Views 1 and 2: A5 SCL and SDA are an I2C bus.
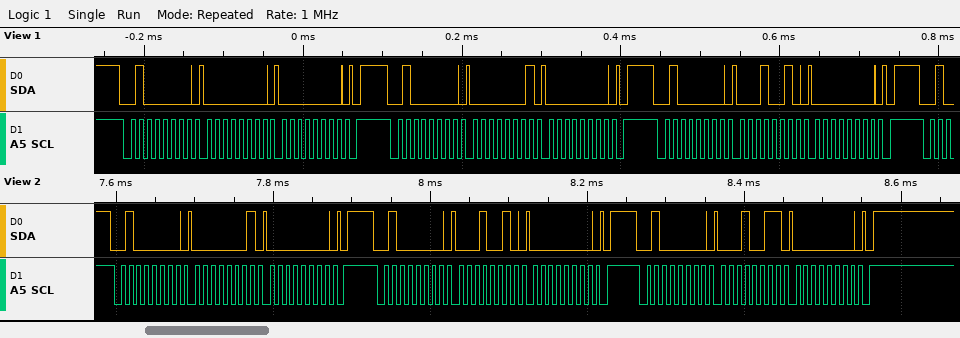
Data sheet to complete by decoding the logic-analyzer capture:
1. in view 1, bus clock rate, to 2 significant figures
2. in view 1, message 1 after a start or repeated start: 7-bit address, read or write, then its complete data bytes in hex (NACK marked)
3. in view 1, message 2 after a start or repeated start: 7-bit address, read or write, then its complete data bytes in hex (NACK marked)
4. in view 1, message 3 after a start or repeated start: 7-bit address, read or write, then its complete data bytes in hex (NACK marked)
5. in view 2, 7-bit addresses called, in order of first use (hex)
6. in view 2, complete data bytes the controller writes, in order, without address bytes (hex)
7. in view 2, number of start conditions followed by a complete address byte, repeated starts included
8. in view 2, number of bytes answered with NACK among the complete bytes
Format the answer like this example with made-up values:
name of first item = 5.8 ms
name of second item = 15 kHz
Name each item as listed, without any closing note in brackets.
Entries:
in view 1, bus clock rate, to 2 significant figures = 100 kHz
in view 1, message 1 after a start or repeated start: 7-bit address, read or write, then its complete data bytes in hex = 0x20 write: 00 00
in view 1, message 2 after a start or repeated start: 7-bit address, read or write, then its complete data bytes in hex = 0x20 write: 01 00
in view 1, message 3 after a start or repeated start: 7-bit address, read or write, then its complete data bytes in hex = 0x20 write: 12 00
in view 2, 7-bit addresses called, in order of first use = 0x20
in view 2, complete data bytes the controller writes, in order, without address bytes = 01 00 12 00 13 00
in view 2, number of start conditions followed by a complete address byte, repeated starts included = 3
in view 2, number of bytes answered with NACK among the complete bytes = 0
